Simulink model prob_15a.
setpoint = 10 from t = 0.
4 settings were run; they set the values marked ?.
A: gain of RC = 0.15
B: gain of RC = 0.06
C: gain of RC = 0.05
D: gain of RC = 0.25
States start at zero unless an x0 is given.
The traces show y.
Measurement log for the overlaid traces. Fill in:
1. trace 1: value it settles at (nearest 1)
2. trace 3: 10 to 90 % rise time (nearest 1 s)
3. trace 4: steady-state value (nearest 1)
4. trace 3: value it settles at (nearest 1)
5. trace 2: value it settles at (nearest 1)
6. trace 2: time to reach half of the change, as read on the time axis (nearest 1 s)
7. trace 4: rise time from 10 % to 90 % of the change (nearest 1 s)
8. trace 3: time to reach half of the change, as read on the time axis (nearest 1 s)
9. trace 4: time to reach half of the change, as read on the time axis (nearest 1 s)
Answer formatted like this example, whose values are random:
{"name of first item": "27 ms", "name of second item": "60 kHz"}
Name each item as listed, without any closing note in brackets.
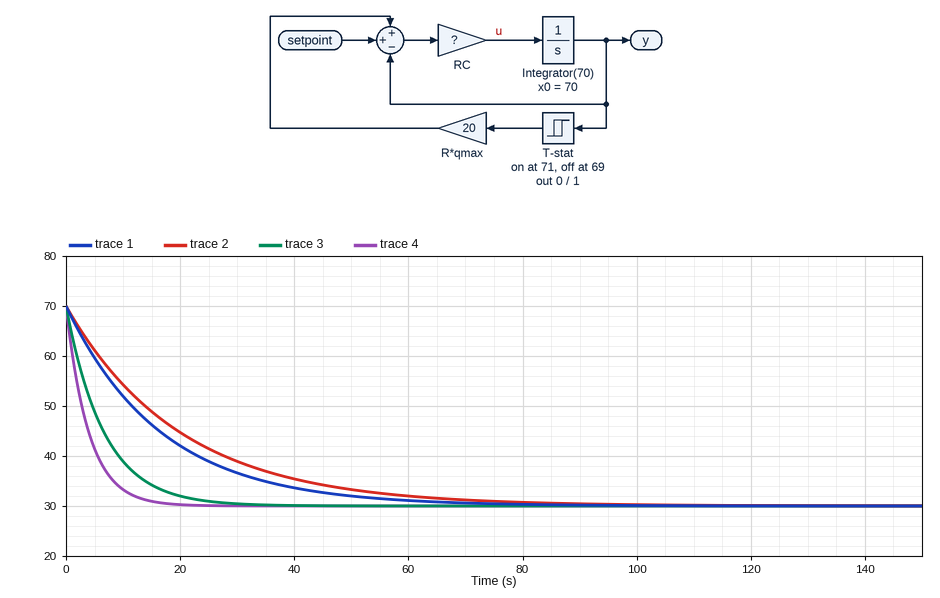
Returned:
{"trace 1: value it settles at": "30", "trace 3: 10 to 90 % rise time": "15 s", "trace 4: steady-state value": "30", "trace 3: value it settles at": "30", "trace 2: value it settles at": "30", "trace 2: time to reach half of the change, as read on the time axis": "14 s", "trace 4: rise time from 10 % to 90 % of the change": "9 s", "trace 3: time to reach half of the change, as read on the time axis": "5 s", "trace 4: time to reach half of the change, as read on the time axis": "3 s"}
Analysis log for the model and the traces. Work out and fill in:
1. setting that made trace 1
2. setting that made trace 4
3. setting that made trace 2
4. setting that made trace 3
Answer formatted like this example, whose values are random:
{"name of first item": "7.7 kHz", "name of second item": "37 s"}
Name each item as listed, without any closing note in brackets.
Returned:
{"setting that made trace 1": "B", "setting that made trace 4": "D", "setting that made trace 2": "C", "setting that made trace 3": "A"}
